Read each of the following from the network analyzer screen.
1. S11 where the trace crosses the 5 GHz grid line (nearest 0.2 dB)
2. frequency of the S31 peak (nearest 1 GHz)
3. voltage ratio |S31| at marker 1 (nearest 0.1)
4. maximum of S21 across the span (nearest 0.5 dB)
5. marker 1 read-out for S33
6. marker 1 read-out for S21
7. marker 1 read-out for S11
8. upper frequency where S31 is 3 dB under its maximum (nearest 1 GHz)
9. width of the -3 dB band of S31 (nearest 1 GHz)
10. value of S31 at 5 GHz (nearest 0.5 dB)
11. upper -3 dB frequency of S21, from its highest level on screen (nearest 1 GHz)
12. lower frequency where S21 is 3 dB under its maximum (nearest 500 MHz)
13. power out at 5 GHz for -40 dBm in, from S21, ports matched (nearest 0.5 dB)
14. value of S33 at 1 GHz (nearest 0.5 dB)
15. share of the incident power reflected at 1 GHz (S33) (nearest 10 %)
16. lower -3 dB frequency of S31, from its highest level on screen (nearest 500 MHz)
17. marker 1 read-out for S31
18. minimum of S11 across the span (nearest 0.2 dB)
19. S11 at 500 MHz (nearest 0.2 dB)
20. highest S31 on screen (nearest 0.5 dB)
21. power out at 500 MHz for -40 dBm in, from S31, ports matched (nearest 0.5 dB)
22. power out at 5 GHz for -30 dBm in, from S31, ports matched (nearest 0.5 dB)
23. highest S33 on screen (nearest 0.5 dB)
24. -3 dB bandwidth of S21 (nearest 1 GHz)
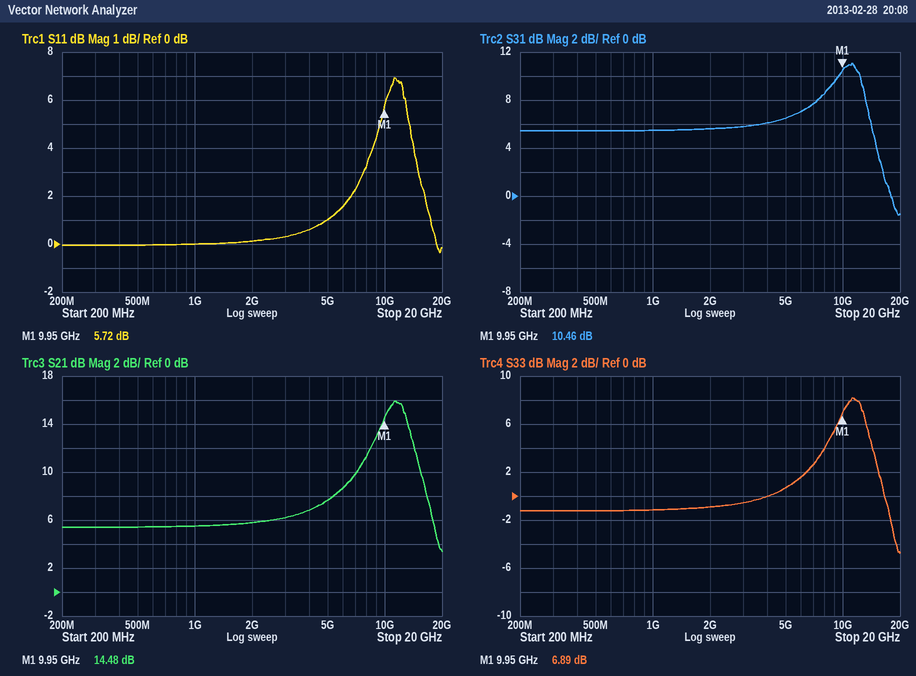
1.0 dB
11 GHz
3.3
16.0 dB
6.89 dB
14.48 dB
5.72 dB
13 GHz
6 GHz
6.5 dB
14 GHz
9.0 GHz
-32.5 dBm
-1.0 dB
80 %
7.5 GHz
10.46 dB
-0.4 dB
0.0 dB
11.0 dB
-34.5 dBm
-23.5 dBm
8.0 dB
5 GHz
